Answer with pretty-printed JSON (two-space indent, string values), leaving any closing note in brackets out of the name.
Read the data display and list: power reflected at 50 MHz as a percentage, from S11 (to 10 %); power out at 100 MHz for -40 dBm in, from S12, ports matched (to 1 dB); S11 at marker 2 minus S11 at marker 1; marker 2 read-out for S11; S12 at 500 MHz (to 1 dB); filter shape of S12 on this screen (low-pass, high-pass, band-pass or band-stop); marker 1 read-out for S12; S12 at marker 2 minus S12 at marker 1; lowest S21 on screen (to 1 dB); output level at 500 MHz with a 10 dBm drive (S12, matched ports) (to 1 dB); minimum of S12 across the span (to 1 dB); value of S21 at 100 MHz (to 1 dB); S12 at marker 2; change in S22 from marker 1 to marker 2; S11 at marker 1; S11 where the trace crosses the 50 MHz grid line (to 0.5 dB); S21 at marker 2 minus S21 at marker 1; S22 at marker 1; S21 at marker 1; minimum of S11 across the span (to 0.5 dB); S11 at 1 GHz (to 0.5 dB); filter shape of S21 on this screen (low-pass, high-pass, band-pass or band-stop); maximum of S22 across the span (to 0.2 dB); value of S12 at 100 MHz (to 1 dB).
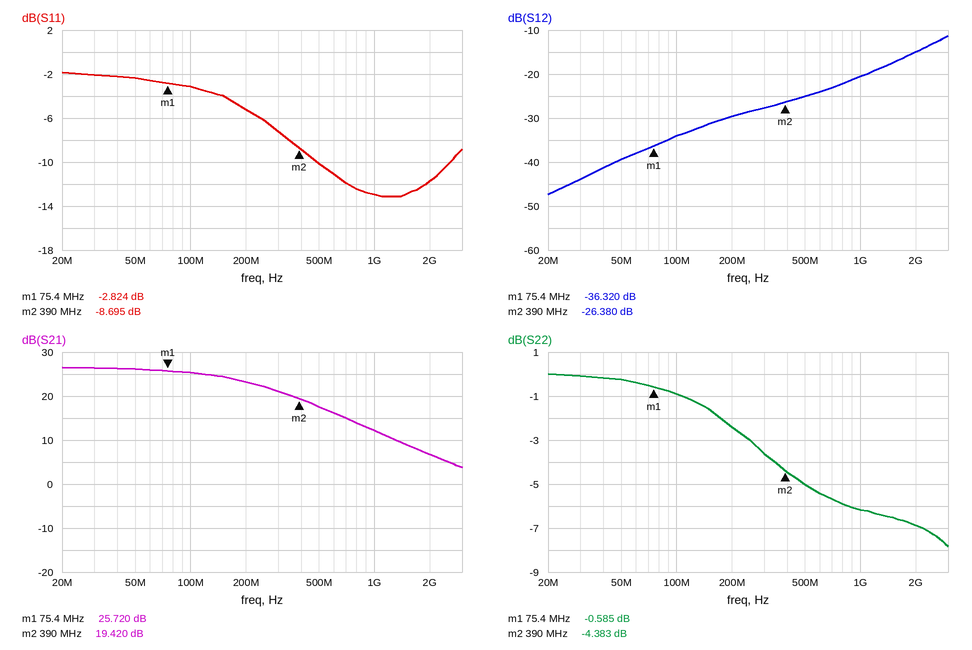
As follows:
{
  "power reflected at 50 MHz as a percentage, from S11": "60 %",
  "power out at 100 MHz for -40 dBm in, from S12, ports matched": "-74 dBm",
  "S11 at marker 2 minus S11 at marker 1": "-5.871 dB",
  "marker 2 read-out for S11": "-8.695 dB",
  "S12 at 500 MHz": "-25 dB",
  "filter shape of S12 on this screen": "high-pass",
  "marker 1 read-out for S12": "-36.320 dB",
  "S12 at marker 2 minus S12 at marker 1": "9.940 dB",
  "lowest S21 on screen": "4 dB",
  "output level at 500 MHz with a 10 dBm drive (S12, matched ports)": "-15 dBm",
  "minimum of S12 across the span": "-47 dB",
  "value of S21 at 100 MHz": "25 dB",
  "S12 at marker 2": "-26.380 dB",
  "change in S22 from marker 1 to marker 2": "-3.798 dB",
  "S11 at marker 1": "-2.824 dB",
  "S11 where the trace crosses the 50 MHz grid line": "-2.5 dB",
  "S21 at marker 2 minus S21 at marker 1": "-6.300 dB",
  "S22 at marker 1": "-0.585 dB",
  "S21 at marker 1": "25.720 dB",
  "minimum of S11 across the span": "-13.0 dB",
  "S11 at 1 GHz": "-13.0 dB",
  "filter shape of S21 on this screen": "low-pass",
  "maximum of S22 across the span": "0.0 dB",
  "value of S12 at 100 MHz": "-34 dB"
}
